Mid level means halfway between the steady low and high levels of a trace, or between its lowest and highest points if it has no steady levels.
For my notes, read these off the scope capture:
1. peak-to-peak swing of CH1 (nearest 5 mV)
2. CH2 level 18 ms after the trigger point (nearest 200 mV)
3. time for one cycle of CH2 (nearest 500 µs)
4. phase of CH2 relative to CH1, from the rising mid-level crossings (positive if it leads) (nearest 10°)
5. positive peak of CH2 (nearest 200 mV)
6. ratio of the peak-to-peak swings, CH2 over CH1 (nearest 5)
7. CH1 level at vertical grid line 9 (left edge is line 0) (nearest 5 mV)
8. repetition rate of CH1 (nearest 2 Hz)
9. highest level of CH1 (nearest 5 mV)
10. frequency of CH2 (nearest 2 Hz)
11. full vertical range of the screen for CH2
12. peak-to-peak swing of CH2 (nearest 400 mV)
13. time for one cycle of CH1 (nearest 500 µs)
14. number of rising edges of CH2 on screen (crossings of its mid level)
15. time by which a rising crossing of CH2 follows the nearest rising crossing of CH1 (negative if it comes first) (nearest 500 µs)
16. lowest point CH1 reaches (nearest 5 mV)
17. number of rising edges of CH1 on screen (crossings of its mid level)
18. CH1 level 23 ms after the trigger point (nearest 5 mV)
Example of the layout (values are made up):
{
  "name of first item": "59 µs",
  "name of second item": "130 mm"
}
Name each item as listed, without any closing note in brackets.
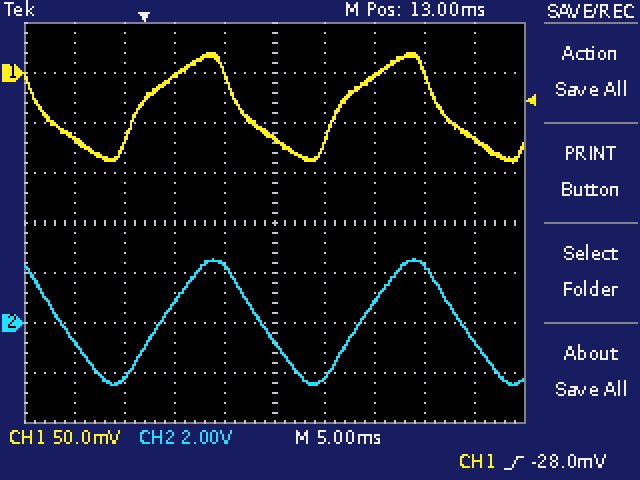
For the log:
{
  "peak-to-peak swing of CH1": "110 mV",
  "CH2 level 18 ms after the trigger point": "-2.2 V",
  "time for one cycle of CH2": "20.0 ms",
  "phase of CH2 relative to CH1, from the rising mid-level crossings (positive if it leads)": "-40°",
  "positive peak of CH2": "2.6 V",
  "ratio of the peak-to-peak swings, CH2 over CH1": "45",
  "CH1 level at vertical grid line 9 (left edge is line 0)": "-65 mV",
  "repetition rate of CH1": "50 Hz",
  "highest level of CH1": "20 mV",
  "frequency of CH2": "50 Hz",
  "full vertical range of the screen for CH2": "16 V",
  "peak-to-peak swing of CH2": "5.2 V",
  "time for one cycle of CH1": "20.0 ms",
  "number of rising edges of CH2 on screen": "2",
  "time by which a rising crossing of CH2 follows the nearest rising crossing of CH1 (negative if it comes first)": "+2.0 ms",
  "lowest point CH1 reaches": "-90 mV",
  "number of rising edges of CH1 on screen": "2",
  "CH1 level 23 ms after the trigger point": "-5 mV"
}
